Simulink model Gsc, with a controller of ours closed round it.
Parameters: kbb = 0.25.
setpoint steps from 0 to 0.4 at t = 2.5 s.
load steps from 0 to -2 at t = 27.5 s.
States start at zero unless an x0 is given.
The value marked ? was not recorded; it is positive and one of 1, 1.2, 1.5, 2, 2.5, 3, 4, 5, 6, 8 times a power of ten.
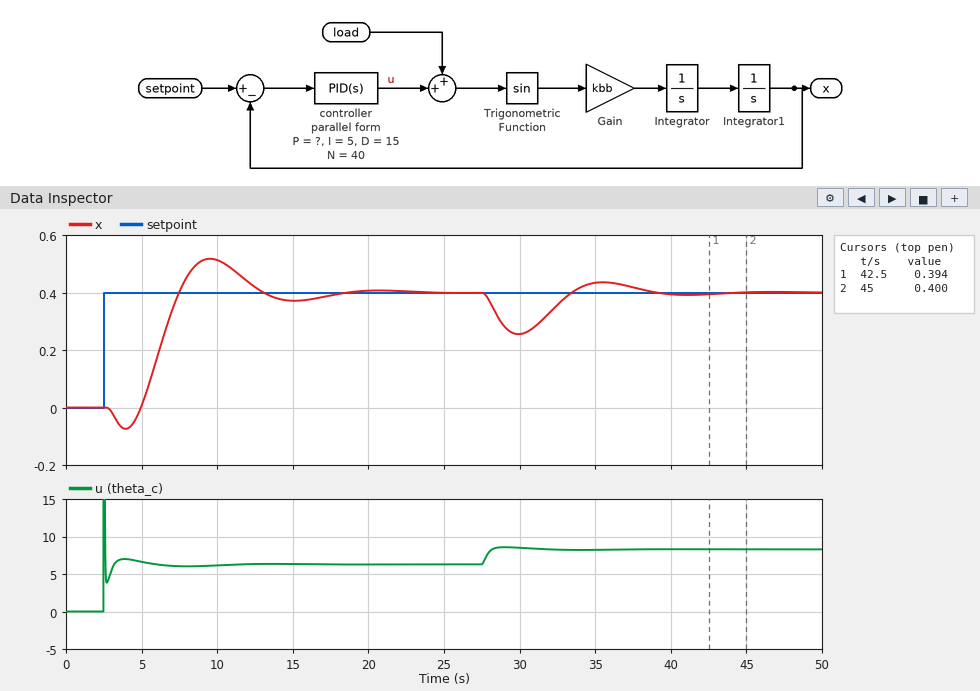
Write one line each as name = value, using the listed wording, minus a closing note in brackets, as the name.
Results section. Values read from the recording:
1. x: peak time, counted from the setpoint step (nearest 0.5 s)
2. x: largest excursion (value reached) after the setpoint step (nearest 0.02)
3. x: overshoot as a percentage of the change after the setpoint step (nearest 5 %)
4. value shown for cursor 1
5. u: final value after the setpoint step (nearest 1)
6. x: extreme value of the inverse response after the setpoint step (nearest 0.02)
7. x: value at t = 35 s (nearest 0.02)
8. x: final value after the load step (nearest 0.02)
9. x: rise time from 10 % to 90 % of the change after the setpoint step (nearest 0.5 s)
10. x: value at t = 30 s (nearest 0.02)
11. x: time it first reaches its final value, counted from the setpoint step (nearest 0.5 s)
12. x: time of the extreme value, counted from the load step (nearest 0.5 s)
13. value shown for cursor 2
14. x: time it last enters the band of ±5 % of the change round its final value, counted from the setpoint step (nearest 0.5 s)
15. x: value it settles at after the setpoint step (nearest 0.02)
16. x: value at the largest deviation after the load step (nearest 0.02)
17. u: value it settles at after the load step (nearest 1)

x: peak time, counted from the setpoint step = 7.0 s
x: largest excursion (value reached) after the setpoint step = 0.52
x: overshoot as a percentage of the change after the setpoint step = 30 %
value shown for cursor 1 = 0.394
u: final value after the setpoint step = 6
x: extreme value of the inverse response after the setpoint step = -0.08
x: value at t = 35 s = 0.44
x: final value after the load step = 0.40
x: rise time from 10 % to 90 % of the change after the setpoint step = 2.0 s
x: value at t = 30 s = 0.26
x: time it first reaches its final value, counted from the setpoint step = 5.0 s
x: time of the extreme value, counted from the load step = 2.5 s
value shown for cursor 2 = 0.400
x: time it last enters the band of ±5 % of the change round its final value, counted from the setpoint step = 14.0 s
x: value it settles at after the setpoint step = 0.40
x: value at the largest deviation after the load step = 0.26
u: value it settles at after the load step = 8
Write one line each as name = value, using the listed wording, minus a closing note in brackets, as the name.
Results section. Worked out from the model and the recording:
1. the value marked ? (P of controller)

the value marked ? = 8
